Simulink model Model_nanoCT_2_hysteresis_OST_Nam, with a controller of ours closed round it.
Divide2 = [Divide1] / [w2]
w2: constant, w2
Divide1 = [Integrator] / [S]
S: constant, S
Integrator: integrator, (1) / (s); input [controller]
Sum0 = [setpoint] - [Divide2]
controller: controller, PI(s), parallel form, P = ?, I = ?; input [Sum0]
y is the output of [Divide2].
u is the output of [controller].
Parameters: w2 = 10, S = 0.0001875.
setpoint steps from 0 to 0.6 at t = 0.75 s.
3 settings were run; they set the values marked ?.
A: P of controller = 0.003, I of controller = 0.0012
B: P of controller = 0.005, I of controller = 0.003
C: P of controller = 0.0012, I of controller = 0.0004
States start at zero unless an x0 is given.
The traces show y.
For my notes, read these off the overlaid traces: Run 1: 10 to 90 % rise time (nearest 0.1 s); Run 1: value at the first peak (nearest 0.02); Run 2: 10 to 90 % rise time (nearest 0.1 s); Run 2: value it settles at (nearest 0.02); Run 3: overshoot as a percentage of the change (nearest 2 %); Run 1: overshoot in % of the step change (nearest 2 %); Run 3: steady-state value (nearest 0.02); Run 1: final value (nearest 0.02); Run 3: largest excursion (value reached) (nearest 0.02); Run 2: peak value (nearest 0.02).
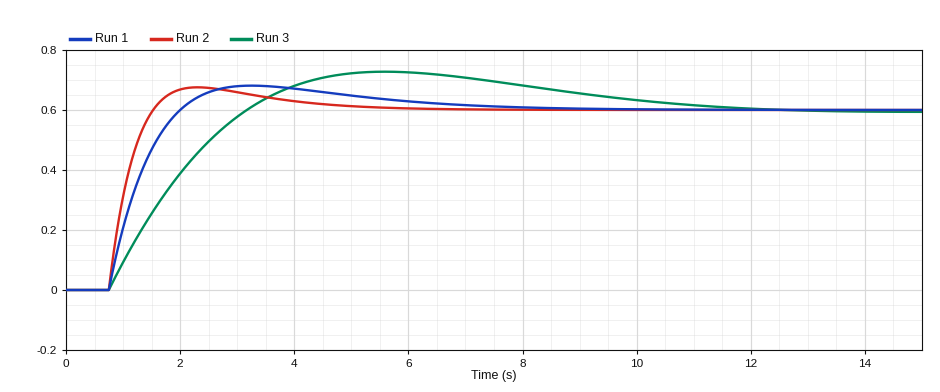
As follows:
0.9 s
0.68
0.6 s
0.60
22 %
14 %
0.60
0.60
0.72
0.68
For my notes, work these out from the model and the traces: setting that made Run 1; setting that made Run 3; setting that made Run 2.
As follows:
A
C
B
